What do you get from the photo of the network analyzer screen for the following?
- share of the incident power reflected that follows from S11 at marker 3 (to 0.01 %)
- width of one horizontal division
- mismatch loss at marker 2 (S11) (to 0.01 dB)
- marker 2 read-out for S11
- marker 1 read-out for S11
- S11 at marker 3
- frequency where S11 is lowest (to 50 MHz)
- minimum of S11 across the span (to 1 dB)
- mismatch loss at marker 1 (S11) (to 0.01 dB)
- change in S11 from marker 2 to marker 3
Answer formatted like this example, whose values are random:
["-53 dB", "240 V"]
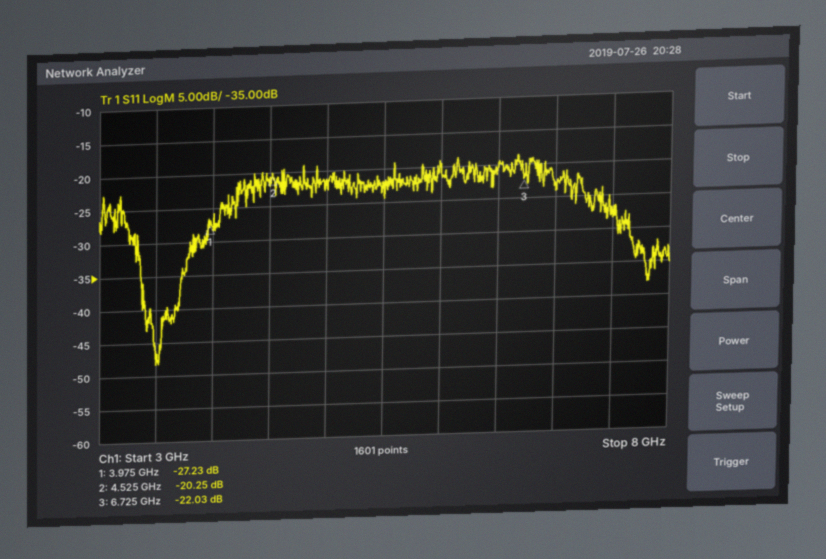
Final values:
["0.63 %", "500 MHz", "0.04 dB", "-20.25 dB", "-27.23 dB", "-22.03 dB", "3.50 GHz", "-48 dB", "0.01 dB", "-1.78 dB"]
